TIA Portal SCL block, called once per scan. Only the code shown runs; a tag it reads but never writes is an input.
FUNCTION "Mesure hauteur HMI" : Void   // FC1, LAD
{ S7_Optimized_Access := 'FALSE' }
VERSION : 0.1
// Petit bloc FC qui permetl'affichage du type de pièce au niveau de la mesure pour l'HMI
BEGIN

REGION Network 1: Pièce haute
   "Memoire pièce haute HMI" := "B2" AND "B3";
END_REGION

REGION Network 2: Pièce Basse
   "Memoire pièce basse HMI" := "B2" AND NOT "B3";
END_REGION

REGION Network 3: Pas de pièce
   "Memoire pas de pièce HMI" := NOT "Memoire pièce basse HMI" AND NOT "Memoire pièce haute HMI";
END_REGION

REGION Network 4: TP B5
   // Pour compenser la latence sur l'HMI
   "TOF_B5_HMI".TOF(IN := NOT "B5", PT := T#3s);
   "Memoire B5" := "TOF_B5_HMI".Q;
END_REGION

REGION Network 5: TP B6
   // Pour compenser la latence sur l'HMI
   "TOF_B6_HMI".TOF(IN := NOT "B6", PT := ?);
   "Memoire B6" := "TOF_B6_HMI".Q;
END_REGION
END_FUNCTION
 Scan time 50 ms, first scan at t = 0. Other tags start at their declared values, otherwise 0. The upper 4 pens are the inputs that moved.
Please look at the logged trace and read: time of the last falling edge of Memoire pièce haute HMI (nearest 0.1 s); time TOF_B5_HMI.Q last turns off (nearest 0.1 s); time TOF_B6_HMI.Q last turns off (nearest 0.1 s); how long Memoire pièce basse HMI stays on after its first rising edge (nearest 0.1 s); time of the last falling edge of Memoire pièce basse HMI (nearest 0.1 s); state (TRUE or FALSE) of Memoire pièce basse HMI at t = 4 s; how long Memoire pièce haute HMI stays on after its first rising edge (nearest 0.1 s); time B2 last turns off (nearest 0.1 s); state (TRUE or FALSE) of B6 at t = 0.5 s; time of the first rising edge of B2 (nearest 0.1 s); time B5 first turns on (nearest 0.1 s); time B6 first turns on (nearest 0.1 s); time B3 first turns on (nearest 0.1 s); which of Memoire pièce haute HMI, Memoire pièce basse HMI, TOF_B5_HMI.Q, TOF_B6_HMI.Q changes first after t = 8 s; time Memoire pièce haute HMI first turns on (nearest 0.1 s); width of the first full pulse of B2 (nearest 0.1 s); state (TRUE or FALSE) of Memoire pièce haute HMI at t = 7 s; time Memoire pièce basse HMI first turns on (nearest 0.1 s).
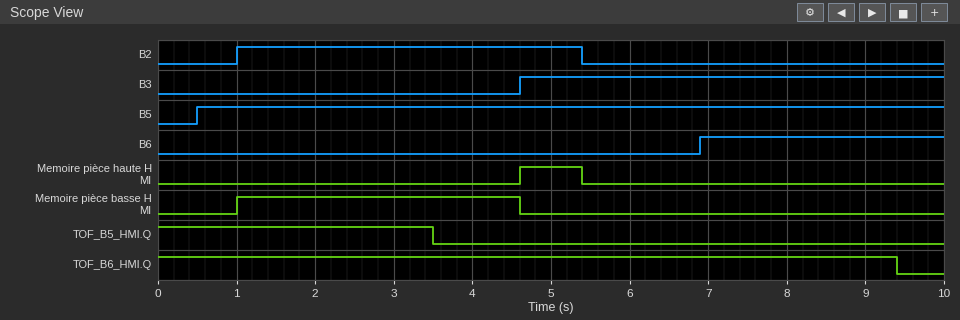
5.4 s
3.5 s
9.4 s
3.6 s
4.6 s
TRUE
0.8 s
5.4 s
FALSE
1.0 s
0.5 s
6.9 s
4.6 s
TOF_B6_HMI.Q
4.6 s
4.4 s
FALSE
1.0 s
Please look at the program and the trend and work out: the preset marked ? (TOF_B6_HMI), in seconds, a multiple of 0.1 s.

2.5 s
